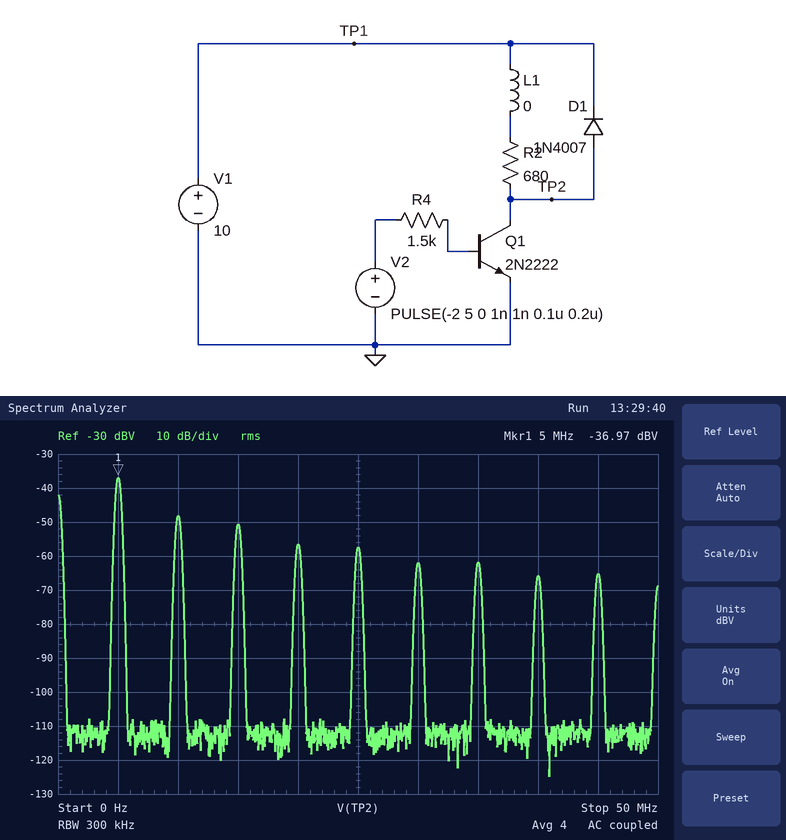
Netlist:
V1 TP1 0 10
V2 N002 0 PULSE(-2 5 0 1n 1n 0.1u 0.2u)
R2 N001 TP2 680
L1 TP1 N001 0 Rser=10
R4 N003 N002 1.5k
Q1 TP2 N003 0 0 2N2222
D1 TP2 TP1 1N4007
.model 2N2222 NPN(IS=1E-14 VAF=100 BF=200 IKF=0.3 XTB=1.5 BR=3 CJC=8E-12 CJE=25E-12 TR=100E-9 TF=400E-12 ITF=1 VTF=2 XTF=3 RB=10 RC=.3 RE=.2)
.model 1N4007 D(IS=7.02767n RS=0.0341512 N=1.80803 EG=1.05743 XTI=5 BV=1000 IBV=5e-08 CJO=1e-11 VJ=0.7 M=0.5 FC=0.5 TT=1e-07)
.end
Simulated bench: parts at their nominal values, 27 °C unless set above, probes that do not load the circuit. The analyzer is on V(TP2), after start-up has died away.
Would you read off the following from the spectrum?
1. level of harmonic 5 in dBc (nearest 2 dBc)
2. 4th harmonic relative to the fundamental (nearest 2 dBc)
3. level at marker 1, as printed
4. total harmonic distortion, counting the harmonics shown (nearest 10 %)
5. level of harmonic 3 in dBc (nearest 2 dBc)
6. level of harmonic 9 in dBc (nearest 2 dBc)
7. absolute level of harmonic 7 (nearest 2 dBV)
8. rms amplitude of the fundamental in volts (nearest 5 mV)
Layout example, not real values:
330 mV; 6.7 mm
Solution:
-20 dBc; -20 dBc; -36.97 dBV; 40 %; -14 dBc; -28 dBc; -62 dBV; 15 mV
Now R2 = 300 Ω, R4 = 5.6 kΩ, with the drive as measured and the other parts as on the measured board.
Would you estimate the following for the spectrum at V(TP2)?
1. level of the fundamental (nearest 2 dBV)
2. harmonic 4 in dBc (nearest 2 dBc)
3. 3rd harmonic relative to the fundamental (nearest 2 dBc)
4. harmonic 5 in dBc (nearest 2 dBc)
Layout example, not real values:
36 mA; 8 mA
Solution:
6 dBV; -24 dBc; -26 dBc; -30 dBc
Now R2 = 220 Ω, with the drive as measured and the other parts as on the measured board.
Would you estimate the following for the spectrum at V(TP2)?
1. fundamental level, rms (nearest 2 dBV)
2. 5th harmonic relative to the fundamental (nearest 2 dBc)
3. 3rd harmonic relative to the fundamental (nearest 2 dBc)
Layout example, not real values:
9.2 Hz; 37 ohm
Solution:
-6 dBV; -4 dBc; -2 dBc
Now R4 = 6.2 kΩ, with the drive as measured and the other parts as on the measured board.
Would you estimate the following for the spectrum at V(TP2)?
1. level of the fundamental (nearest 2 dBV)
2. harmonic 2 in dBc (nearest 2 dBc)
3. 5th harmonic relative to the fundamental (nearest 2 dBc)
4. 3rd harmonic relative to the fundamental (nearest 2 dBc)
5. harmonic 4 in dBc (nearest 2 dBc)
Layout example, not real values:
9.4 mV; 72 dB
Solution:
-14 dBV; -2 dBc; -10 dBc; -4 dBc; -6 dBc
